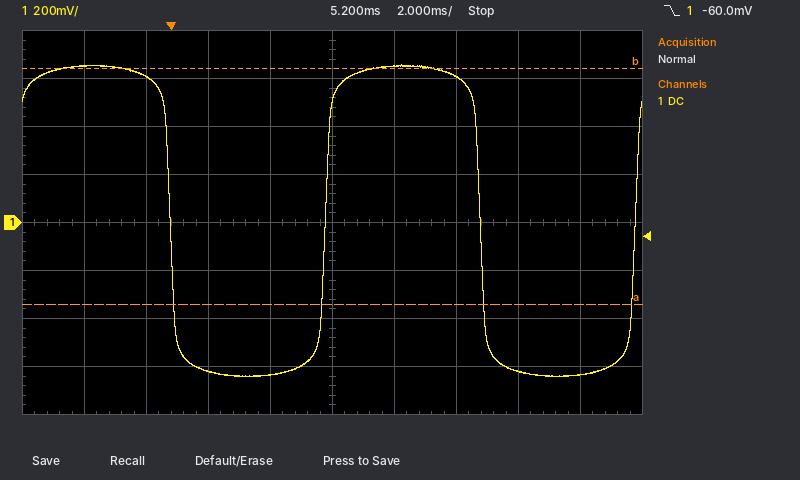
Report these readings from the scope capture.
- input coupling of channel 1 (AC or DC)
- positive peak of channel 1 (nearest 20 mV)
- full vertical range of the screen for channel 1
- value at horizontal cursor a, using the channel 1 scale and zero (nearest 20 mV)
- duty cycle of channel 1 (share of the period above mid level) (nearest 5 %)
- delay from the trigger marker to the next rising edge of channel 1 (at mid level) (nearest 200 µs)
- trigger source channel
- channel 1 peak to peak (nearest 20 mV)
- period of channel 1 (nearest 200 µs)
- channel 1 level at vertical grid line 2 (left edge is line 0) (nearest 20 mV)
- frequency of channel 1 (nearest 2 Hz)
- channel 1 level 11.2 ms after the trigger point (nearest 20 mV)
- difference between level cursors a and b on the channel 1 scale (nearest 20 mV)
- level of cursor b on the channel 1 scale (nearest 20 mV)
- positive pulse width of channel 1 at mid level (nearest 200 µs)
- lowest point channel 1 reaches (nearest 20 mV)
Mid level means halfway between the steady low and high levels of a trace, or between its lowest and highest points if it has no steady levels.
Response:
DC
660 mV
1.6 V
-340 mV
50 %
5.0 ms
channel 1
1.30 V
10.0 ms
600 mV
100 Hz
-620 mV
980 mV
640 mV
5.0 ms
-640 mV
